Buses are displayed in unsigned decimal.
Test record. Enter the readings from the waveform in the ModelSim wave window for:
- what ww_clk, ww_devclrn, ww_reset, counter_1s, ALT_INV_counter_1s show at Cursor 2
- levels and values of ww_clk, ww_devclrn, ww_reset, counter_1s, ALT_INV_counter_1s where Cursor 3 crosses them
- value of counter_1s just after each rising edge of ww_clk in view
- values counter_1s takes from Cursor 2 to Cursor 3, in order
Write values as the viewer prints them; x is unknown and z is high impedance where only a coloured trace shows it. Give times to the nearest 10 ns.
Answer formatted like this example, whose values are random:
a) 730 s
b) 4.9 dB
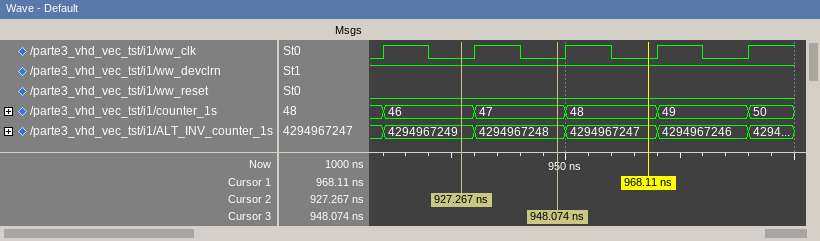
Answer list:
a) ww_clk=0, ww_devclrn=1, ww_reset=0, counter_1s=46, ALT_INV_counter_1s=4294967249
b) ww_clk=0, ww_devclrn=1, ww_reset=0, counter_1s=47, ALT_INV_counter_1s=4294967248
c) 46, 47, 48, 49, 50
d) 46, 47
